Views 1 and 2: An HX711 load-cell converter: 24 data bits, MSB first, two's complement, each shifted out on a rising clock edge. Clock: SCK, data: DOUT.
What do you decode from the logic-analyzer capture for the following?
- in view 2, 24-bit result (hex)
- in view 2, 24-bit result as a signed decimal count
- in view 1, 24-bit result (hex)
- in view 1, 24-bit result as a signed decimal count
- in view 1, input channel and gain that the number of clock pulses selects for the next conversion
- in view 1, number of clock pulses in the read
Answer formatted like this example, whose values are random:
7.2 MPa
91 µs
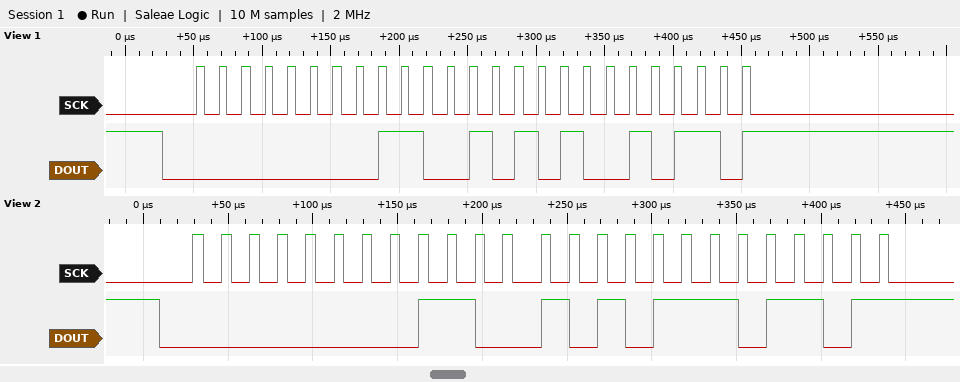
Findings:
0x00CAED
51949
0x00CA96
51862
channel A, gain 128
25
